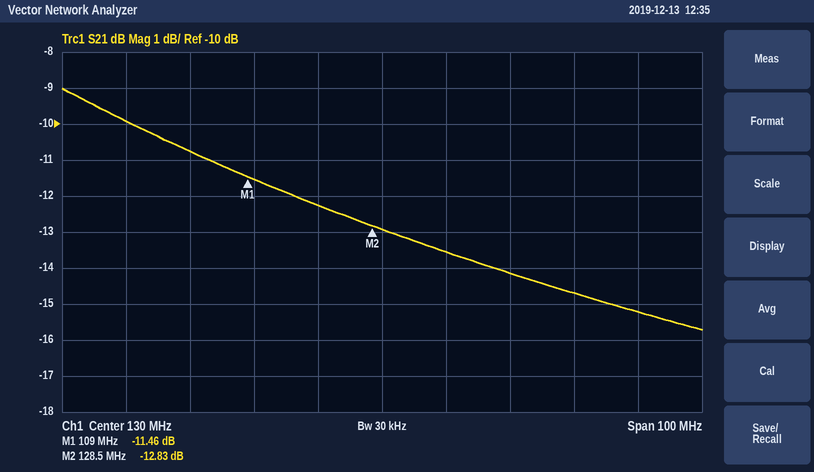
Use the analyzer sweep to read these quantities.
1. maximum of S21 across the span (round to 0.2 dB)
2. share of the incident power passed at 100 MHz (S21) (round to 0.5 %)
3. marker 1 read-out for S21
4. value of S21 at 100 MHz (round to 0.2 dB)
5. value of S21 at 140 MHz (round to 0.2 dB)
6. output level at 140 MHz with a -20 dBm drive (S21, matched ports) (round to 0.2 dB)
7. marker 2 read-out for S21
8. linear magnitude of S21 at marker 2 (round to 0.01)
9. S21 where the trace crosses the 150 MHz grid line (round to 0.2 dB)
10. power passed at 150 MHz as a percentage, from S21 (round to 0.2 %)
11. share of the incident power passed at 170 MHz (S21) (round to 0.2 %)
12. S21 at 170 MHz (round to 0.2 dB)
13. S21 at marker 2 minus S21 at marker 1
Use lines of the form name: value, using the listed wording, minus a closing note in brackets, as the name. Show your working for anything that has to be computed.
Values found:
maximum of S21 across the span: -9.0 dB
share of the incident power passed at 100 MHz (S21): 10^(-10.8/10) ≈ 8.32 %, so 8.5 % to the nearest 0.5 %
marker 1 read-out for S21: -11.46 dB
value of S21 at 100 MHz: -10.8 dB
value of S21 at 140 MHz: -13.6 dB
output level at 140 MHz with a -20 dBm drive (S21, matched ports): -20 dBm + (-13.6 dB) = -33.6 dBm
marker 2 read-out for S21: -12.83 dB
linear magnitude of S21 at marker 2: 10^(-12.83/20) ≈ 0.23
S21 where the trace crosses the 150 MHz grid line: -14.2 dB
power passed at 150 MHz as a percentage, from S21: 10^(-14.2/10) ≈ 3.8 %
share of the incident power passed at 170 MHz (S21): 10^(-15.2/10) ≈ 3.0 %
S21 at 170 MHz: -15.2 dB
S21 at marker 2 minus S21 at marker 1: -12.83 − (-11.46) = -1.37 dB
